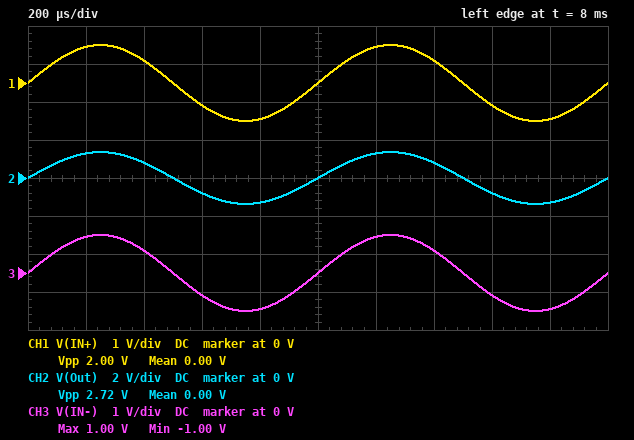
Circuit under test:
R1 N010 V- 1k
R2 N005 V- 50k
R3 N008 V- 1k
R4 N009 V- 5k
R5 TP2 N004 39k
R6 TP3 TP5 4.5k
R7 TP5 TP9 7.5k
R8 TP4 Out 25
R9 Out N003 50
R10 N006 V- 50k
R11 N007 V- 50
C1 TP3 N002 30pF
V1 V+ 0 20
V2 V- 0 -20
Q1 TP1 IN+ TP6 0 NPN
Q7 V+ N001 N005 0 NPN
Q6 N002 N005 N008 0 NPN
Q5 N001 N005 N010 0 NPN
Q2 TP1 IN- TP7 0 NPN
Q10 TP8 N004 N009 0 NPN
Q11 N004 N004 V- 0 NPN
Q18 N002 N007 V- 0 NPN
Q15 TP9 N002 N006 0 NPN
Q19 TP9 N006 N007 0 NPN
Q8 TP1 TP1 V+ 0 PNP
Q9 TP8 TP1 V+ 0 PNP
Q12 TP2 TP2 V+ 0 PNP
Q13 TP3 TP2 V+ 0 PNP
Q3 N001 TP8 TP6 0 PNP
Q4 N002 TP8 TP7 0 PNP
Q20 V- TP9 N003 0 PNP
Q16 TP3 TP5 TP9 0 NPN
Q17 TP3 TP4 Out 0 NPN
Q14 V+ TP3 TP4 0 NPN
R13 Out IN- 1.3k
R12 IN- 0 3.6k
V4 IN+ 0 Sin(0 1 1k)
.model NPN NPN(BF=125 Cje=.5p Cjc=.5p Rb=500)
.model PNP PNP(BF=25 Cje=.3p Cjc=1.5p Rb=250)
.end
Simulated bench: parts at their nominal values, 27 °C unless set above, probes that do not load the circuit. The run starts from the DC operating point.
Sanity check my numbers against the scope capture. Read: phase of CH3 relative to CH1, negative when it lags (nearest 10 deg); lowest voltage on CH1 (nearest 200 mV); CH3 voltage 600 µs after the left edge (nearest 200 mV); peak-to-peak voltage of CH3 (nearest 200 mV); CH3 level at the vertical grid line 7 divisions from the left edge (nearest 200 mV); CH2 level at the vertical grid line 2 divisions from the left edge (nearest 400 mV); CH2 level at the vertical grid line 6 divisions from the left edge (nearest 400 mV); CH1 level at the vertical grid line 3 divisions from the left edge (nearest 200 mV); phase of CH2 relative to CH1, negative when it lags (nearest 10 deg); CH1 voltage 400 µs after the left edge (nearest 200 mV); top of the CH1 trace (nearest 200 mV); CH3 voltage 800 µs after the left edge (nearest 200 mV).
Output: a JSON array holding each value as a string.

["0 deg", "-1.0 V", "-600 mV", "2.0 V", "600 mV", "800 mV", "1.2 V", "-600 mV", "0 deg", "600 mV", "1.0 V", "-1.0 V"]
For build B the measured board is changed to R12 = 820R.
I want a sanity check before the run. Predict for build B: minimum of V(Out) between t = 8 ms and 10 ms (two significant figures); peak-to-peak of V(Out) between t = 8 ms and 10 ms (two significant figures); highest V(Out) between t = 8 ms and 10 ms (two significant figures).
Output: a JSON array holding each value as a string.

["-2.6 V", "5.2 V", "2.6 V"]
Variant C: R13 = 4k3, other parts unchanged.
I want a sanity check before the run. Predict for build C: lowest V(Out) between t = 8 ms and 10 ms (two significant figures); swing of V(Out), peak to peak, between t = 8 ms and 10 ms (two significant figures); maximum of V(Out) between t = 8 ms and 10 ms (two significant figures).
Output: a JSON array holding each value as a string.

["-2.2 V", "4.4 V", "2.2 V"]
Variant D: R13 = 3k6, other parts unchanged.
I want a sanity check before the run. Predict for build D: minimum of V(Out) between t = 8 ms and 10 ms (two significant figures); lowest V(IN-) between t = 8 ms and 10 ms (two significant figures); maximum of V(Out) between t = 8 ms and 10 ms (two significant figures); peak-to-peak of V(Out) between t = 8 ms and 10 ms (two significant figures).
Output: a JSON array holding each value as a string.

["-2.0 V", "-1.0 V", "2.0 V", "4.0 V"]
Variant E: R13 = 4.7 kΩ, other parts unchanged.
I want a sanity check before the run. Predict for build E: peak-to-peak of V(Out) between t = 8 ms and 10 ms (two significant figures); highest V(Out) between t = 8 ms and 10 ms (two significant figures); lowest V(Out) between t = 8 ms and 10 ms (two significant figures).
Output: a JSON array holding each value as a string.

["4.6 V", "2.3 V", "-2.3 V"]
